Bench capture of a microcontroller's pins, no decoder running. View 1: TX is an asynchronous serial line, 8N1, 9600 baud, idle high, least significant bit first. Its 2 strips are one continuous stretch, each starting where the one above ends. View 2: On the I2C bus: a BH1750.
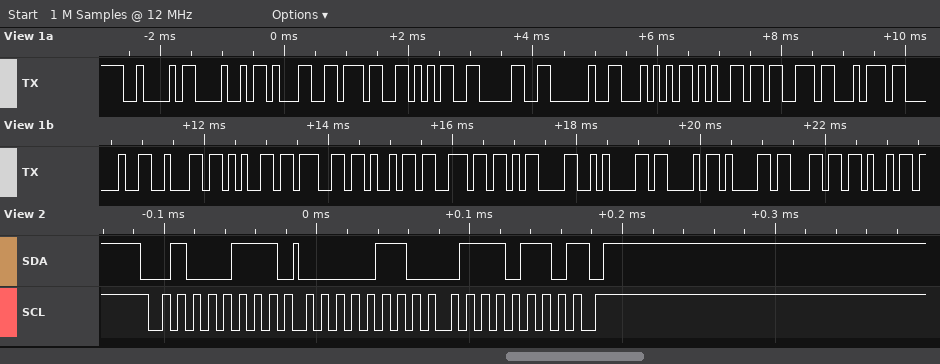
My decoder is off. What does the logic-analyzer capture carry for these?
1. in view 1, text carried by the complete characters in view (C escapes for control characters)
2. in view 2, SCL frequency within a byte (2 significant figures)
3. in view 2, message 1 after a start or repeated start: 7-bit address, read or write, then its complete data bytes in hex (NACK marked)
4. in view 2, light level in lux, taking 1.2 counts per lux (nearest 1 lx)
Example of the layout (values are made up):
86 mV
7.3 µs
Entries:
"BH1750 Test begin\r\nCali"
100 kHz
0x23 read: 06 76 NACK
1378 lx
